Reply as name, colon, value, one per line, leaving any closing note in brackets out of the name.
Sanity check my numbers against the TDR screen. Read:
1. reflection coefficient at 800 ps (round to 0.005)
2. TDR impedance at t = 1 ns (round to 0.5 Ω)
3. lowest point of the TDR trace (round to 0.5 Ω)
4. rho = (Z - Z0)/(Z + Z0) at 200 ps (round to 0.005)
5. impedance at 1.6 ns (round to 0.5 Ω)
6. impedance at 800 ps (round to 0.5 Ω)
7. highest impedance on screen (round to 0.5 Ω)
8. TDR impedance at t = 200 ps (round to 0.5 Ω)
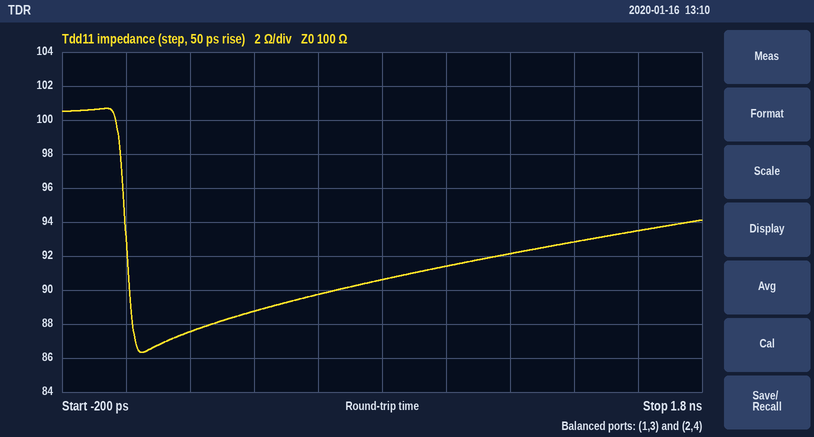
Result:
reflection coefficient at 800 ps: -0.050
TDR impedance at t = 1 ns: 91.5 Ω
lowest point of the TDR trace: 86.5 Ω
rho = (Z - Z0)/(Z + Z0) at 200 ps: -0.065
impedance at 1.6 ns: 93.5 Ω
impedance at 800 ps: 90.5 Ω
highest impedance on screen: 100.5 Ω
TDR impedance at t = 200 ps: 87.5 Ω
